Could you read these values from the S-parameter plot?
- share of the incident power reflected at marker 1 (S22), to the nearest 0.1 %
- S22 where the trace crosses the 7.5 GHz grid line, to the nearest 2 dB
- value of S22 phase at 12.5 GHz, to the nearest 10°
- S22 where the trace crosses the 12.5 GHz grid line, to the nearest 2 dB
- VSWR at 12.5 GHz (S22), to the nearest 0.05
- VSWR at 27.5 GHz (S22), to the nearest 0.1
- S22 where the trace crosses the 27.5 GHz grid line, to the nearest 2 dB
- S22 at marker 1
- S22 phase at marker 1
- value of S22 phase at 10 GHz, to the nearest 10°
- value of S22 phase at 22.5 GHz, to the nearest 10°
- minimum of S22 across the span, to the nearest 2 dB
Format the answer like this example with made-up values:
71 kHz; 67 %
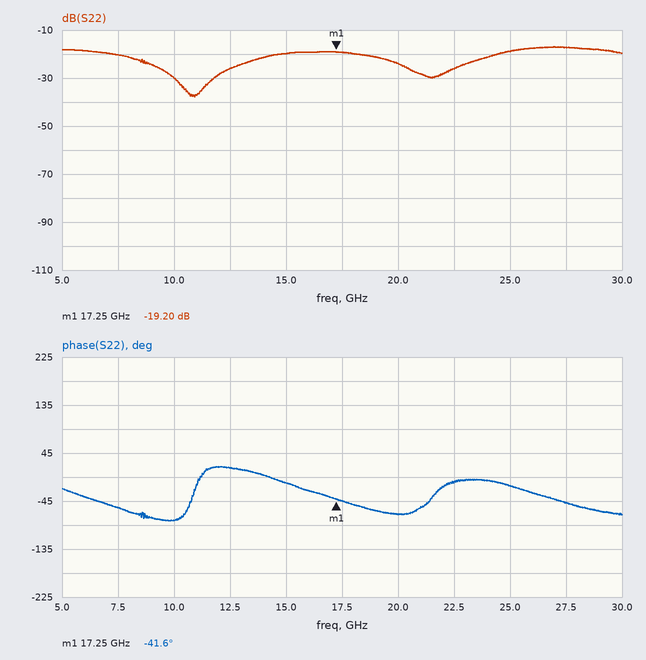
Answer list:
1.2 %; -20 dB; 20°; -26 dB; 1.10; 1.3; -18 dB; -19.20 dB; -41.6°; -80°; -10°; -38 dB
